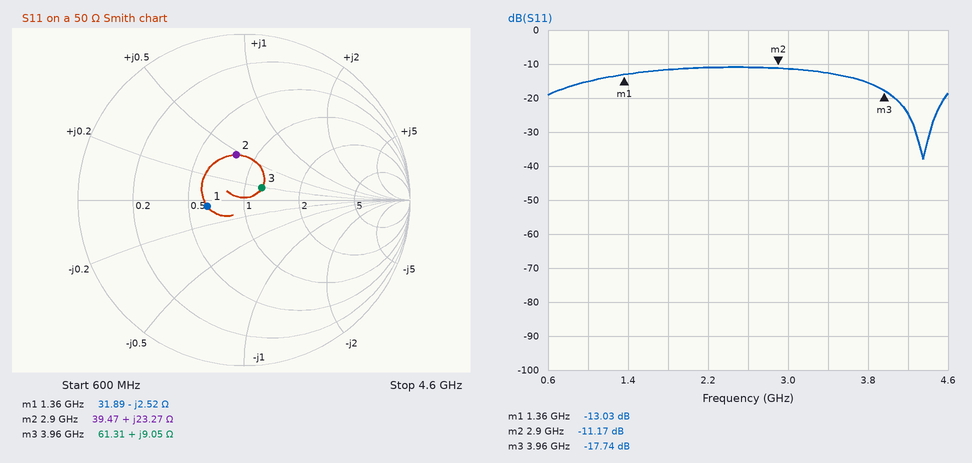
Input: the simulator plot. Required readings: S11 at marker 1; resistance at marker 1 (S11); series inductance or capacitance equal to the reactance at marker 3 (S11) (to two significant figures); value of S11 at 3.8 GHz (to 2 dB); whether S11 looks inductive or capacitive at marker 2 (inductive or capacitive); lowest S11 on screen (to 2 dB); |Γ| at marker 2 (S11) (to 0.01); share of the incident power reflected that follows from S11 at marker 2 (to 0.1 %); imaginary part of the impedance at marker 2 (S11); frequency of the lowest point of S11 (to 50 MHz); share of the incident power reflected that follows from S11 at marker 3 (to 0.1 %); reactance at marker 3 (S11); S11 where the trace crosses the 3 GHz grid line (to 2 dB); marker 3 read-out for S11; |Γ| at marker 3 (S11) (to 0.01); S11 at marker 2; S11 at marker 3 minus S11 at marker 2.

-13.03 dB
31.89 Ω
360 pH
-16 dB
inductive
-38 dB
0.28
7.6 %
+23.27 Ω
4.35 GHz
1.7 %
+9.05 Ω
-12 dB
-17.74 dB
0.13
-11.17 dB
-6.57 dB
